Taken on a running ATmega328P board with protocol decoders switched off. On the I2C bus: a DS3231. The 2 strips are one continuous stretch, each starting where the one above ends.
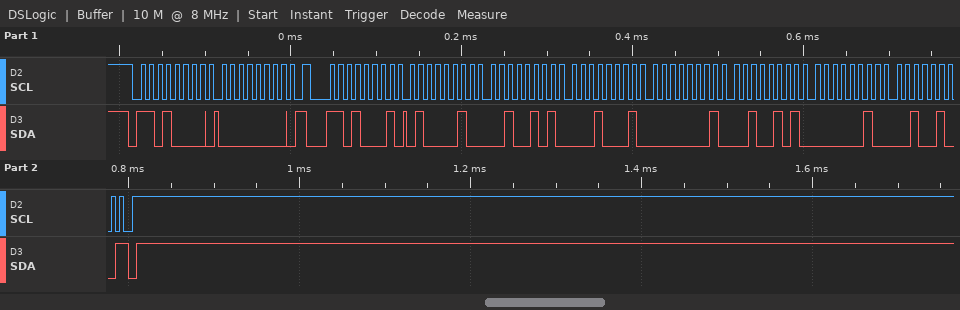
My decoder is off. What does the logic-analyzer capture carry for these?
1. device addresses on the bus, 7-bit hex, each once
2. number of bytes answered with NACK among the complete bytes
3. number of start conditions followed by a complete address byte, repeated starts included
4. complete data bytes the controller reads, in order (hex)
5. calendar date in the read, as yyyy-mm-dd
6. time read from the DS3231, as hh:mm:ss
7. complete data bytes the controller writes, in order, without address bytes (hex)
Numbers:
0x68
1
2
42 25 11 01 25 02 24
2024-02-25
11:25:42
00
